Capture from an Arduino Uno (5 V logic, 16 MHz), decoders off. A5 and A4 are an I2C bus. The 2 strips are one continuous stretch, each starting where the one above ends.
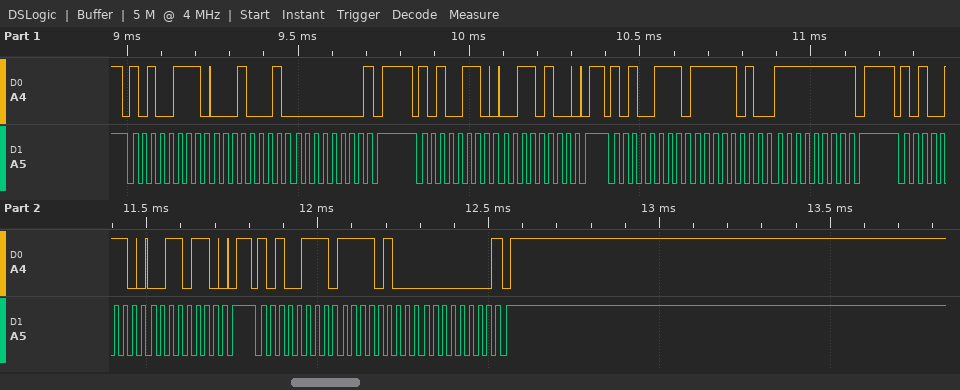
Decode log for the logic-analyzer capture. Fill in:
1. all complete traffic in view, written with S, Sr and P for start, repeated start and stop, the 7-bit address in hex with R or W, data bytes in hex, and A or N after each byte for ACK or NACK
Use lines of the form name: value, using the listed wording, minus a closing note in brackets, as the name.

all complete traffic in view, written with S, Sr and P for start, repeated start and stop, the 7-bit address in hex with R or W, data bytes in hex, and A or N after each byte for ACK or NACK: S 53R A 11 A 00 N P S 53W A 34 A P S 53R A FA A FF N P S 53W A 36 A P S 53R A F4 A 00 N P
